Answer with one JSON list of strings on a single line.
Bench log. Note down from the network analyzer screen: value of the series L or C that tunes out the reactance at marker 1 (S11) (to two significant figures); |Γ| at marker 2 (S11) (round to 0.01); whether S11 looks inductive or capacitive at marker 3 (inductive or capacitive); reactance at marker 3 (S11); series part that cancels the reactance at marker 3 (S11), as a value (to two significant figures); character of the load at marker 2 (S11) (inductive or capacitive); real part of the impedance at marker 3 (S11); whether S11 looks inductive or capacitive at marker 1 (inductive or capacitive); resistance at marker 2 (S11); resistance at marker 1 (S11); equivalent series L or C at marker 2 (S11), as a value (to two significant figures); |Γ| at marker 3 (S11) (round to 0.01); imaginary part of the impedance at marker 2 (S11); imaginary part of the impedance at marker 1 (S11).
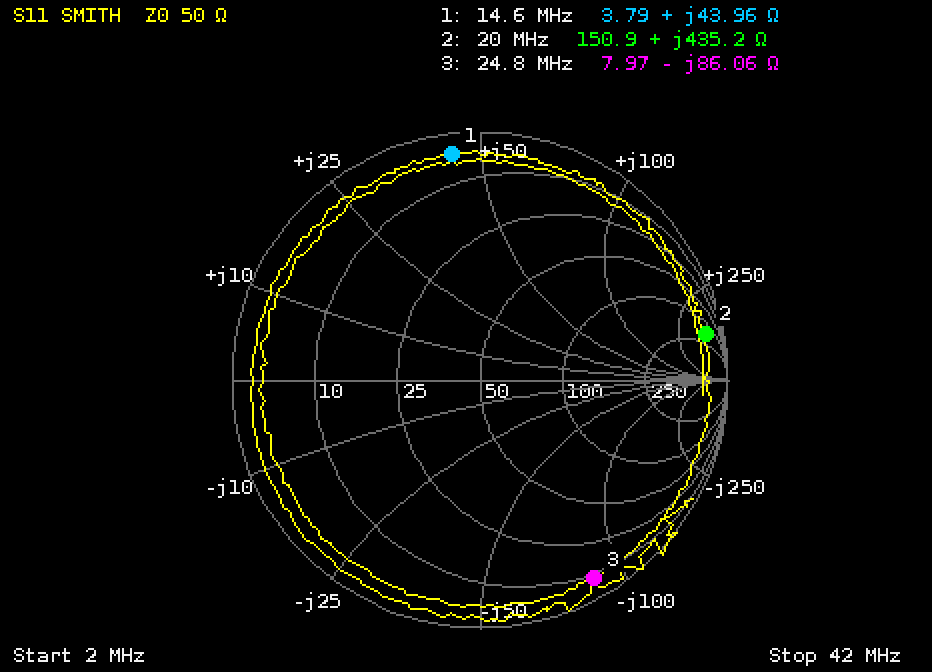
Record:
["250 pF", "0.93", "capacitive", "-86.06 Ω", "550 nH", "inductive", "7.97 Ω", "inductive", "150.9 Ω", "3.79 Ω", "3.5 µH", "0.92", "+435.2 Ω", "+43.96 Ω"]
